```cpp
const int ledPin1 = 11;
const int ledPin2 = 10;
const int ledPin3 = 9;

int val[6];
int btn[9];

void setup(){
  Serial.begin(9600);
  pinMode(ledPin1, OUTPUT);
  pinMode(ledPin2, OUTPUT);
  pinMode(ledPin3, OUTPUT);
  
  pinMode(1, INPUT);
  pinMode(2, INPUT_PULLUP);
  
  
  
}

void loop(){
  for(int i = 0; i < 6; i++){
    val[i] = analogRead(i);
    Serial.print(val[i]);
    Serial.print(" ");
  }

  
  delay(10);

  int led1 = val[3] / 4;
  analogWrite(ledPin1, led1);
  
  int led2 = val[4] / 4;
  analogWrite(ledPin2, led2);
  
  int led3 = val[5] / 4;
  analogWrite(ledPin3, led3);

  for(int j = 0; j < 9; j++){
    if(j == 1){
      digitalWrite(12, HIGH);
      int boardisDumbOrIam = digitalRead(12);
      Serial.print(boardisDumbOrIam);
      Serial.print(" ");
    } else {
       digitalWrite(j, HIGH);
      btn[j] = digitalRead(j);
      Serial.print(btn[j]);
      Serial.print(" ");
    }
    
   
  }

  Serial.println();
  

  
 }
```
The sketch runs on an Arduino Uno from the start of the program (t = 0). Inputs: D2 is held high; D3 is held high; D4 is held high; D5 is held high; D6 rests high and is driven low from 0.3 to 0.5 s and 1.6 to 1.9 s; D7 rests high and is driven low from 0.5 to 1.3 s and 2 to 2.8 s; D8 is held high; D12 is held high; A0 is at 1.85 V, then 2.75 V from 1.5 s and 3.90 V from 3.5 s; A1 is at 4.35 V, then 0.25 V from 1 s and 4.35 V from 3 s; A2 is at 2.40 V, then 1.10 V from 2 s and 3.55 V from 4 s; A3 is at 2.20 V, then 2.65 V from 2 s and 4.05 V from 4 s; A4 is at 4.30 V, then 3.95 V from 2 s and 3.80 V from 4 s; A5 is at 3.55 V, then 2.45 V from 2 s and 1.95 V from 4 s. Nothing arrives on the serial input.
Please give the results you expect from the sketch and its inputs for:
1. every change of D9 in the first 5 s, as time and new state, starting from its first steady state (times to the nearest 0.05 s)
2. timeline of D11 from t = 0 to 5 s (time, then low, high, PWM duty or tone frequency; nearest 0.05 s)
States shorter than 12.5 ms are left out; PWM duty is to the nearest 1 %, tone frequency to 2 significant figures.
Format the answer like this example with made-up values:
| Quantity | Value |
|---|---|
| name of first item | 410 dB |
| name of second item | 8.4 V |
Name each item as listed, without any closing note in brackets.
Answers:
| Quantity | Value |
|---|---|
| every change of D9 in the first 5 s, as time and new state, starting from its first steady state | 0 s PWM 71 %; 2.05 s PWM 49 %; 4.05 s PWM 39 % |
| timeline of D11 from t = 0 to 5 s | 0 s PWM 44 %; 2.05 s PWM 53 %; 4.05 s PWM 81 % |
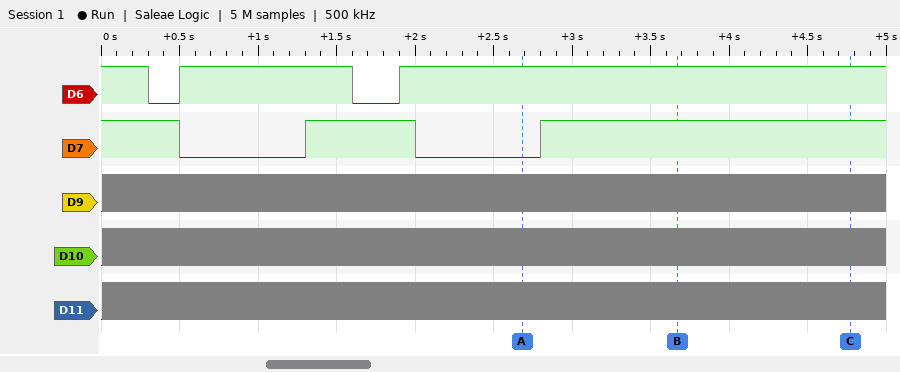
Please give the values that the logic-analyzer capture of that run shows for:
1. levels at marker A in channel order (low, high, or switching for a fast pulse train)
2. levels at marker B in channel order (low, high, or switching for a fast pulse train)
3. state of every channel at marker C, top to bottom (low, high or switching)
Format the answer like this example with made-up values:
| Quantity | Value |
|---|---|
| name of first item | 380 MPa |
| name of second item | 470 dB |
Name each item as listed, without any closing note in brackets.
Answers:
| Quantity | Value |
|---|---|
| levels at marker A in channel order | D6 high, D7 low, D9 switching, D10 switching, D11 switching |
| levels at marker B in channel order | D6 high, D7 high, D9 switching, D10 switching, D11 switching |
| state of every channel at marker C, top to bottom | D6 high, D7 high, D9 switching, D10 switching, D11 switching |
